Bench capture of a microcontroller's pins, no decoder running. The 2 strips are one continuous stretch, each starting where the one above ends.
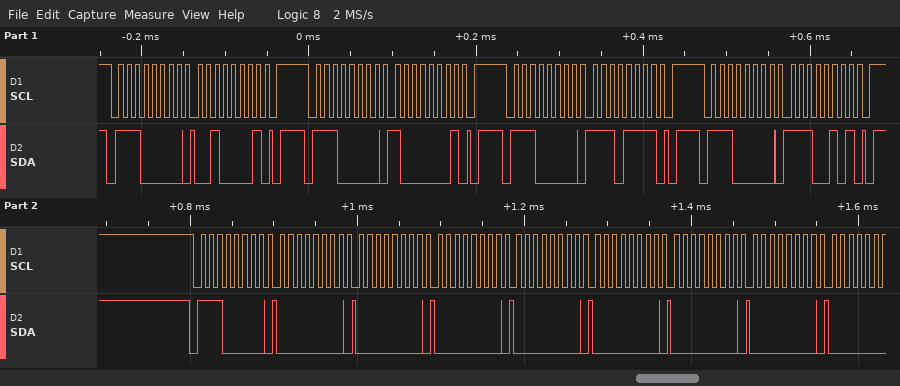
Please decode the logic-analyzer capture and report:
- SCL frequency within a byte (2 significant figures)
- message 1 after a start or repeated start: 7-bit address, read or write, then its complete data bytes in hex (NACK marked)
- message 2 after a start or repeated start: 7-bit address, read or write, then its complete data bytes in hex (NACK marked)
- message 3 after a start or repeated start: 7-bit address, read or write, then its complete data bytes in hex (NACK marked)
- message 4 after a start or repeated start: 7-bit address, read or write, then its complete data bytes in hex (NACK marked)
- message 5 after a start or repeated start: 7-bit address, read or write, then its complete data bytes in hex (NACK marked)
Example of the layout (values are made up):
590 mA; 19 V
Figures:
100 kHz; 0x70 write: 21; 0x70 write: 81; 0x70 write: EF; 0x70 write: E5; 0x70 write: 00 00 00 00 00 00 00
